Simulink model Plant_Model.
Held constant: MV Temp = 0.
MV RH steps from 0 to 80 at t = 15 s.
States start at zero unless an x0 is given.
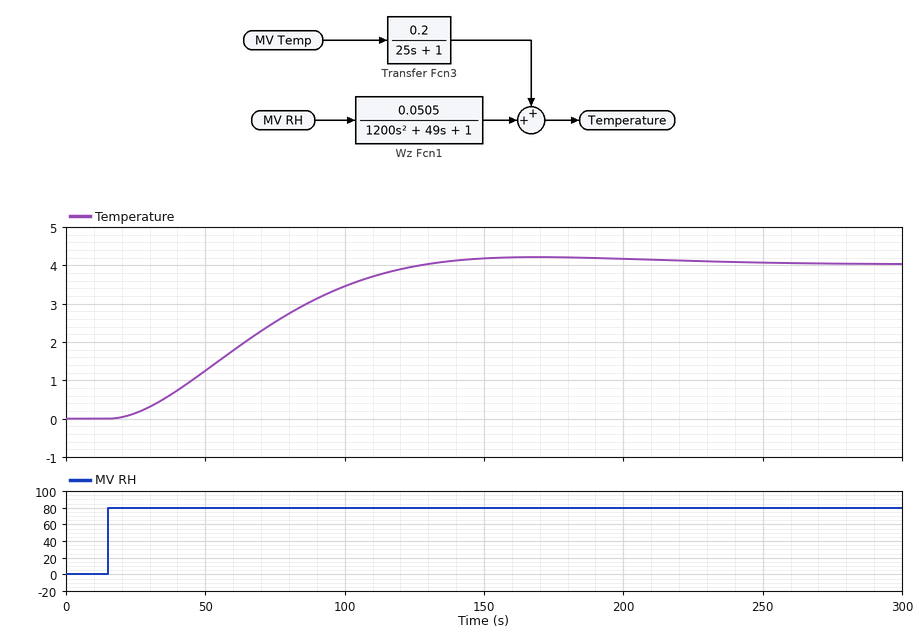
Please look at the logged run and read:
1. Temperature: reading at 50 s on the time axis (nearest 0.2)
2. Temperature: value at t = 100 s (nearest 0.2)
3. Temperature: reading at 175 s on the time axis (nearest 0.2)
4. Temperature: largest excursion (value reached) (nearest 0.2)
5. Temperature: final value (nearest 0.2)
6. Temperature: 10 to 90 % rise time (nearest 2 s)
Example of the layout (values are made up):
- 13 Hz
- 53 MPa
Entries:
- 1.2
- 3.4
- 4.2
- 4.2
- 4.0
- 74 s
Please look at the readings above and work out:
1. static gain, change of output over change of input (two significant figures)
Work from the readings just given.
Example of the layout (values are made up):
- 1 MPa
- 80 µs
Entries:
- 0.050
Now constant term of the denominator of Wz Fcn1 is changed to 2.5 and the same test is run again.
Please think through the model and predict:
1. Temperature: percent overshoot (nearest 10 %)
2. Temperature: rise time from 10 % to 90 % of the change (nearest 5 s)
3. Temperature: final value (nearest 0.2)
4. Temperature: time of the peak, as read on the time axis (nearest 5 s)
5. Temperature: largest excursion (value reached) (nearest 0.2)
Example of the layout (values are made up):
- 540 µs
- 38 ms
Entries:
- 20 %
- 35 s
- 1.6
- 90 s
- 2.0
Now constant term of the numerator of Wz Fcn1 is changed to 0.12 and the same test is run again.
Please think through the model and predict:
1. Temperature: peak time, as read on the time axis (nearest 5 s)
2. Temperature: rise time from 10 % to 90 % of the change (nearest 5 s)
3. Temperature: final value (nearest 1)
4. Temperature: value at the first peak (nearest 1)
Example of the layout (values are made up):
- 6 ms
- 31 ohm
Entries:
- 170 s
- 75 s
- 10
- 10
